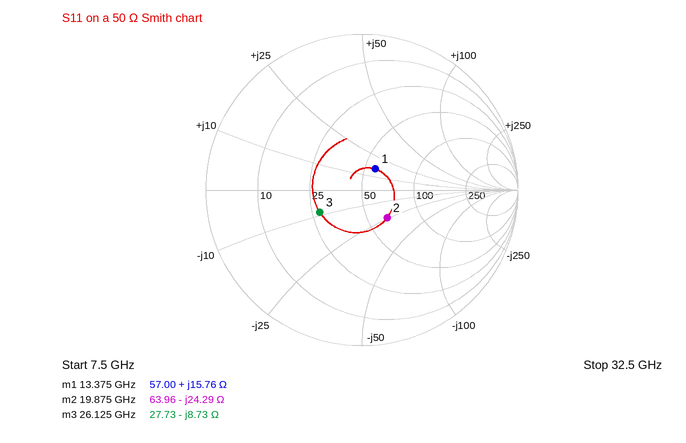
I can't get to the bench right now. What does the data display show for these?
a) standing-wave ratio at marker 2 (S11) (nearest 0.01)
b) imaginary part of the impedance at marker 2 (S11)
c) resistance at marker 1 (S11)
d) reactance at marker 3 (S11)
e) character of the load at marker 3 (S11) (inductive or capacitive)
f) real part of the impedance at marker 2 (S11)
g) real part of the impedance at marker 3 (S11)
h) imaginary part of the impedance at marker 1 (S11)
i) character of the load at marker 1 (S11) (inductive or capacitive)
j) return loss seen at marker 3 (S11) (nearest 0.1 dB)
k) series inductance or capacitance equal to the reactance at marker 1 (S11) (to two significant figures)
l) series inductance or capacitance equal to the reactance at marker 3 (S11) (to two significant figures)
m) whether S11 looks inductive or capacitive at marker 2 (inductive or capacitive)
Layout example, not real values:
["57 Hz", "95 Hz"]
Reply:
["1.63", "-24.29 Ω", "57.00 Ω", "-8.73 Ω", "capacitive", "63.96 Ω", "27.73 Ω", "+15.76 Ω", "inductive", "10.3 dB", "190 pH", "700 fF", "capacitive"]
